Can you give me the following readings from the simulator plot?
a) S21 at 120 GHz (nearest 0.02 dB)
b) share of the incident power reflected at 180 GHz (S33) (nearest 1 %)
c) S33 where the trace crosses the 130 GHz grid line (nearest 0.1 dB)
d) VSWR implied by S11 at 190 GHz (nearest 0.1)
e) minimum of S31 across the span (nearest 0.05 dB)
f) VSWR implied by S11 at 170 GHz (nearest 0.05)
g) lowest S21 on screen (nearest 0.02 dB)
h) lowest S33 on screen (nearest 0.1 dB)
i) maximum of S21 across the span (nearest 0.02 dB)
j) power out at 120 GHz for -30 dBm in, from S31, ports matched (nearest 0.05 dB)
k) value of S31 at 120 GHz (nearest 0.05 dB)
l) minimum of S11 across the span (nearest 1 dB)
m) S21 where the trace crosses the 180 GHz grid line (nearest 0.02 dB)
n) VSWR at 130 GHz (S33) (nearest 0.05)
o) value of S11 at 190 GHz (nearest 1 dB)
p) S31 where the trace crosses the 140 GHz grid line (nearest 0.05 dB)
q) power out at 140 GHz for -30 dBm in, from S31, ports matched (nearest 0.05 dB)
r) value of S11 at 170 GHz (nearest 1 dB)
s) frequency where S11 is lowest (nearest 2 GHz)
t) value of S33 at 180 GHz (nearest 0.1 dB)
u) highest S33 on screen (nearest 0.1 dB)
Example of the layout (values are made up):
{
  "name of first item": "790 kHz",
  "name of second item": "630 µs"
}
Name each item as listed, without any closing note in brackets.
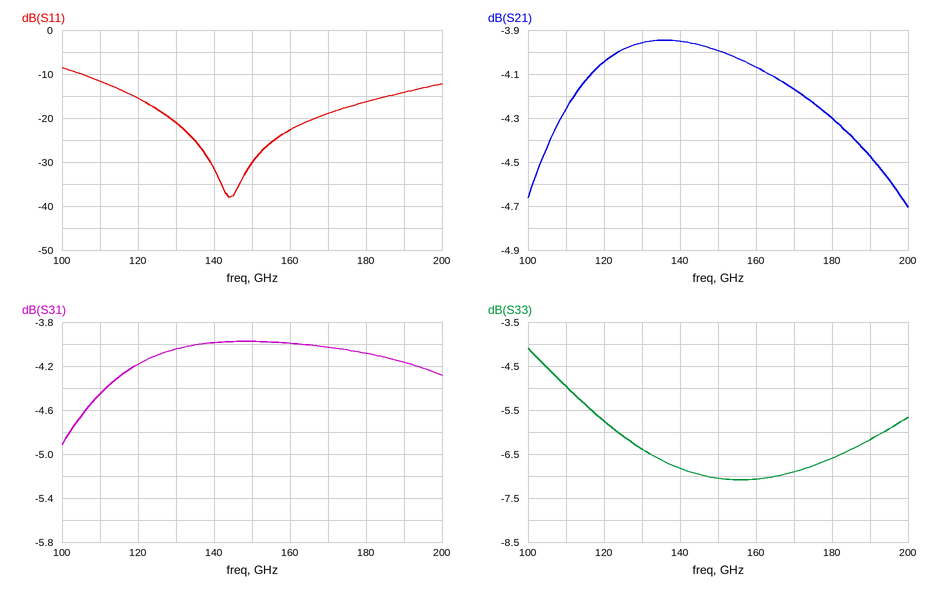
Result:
{
  "S21 at 120 GHz": "-4.04 dB",
  "share of the incident power reflected at 180 GHz (S33)": "22 %",
  "S33 where the trace crosses the 130 GHz grid line": "-6.4 dB",
  "VSWR implied by S11 at 190 GHz": "1.5",
  "minimum of S31 across the span": "-4.90 dB",
  "VSWR implied by S11 at 170 GHz": "1.25",
  "lowest S21 on screen": "-4.70 dB",
  "lowest S33 on screen": "-7.1 dB",
  "maximum of S21 across the span": "-3.94 dB",
  "power out at 120 GHz for -30 dBm in, from S31, ports matched": "-34.20 dBm",
  "value of S31 at 120 GHz": "-4.20 dB",
  "minimum of S11 across the span": "-38 dB",
  "S21 where the trace crosses the 180 GHz grid line": "-4.30 dB",
  "VSWR at 130 GHz (S33)": "2.85",
  "value of S11 at 190 GHz": "-14 dB",
  "S31 where the trace crosses the 140 GHz grid line": "-4.00 dB",
  "power out at 140 GHz for -30 dBm in, from S31, ports matched": "-34.00 dBm",
  "value of S11 at 170 GHz": "-19 dB",
  "frequency where S11 is lowest": "144 GHz",
  "value of S33 at 180 GHz": "-6.6 dB",
  "highest S33 on screen": "-4.1 dB"
}
